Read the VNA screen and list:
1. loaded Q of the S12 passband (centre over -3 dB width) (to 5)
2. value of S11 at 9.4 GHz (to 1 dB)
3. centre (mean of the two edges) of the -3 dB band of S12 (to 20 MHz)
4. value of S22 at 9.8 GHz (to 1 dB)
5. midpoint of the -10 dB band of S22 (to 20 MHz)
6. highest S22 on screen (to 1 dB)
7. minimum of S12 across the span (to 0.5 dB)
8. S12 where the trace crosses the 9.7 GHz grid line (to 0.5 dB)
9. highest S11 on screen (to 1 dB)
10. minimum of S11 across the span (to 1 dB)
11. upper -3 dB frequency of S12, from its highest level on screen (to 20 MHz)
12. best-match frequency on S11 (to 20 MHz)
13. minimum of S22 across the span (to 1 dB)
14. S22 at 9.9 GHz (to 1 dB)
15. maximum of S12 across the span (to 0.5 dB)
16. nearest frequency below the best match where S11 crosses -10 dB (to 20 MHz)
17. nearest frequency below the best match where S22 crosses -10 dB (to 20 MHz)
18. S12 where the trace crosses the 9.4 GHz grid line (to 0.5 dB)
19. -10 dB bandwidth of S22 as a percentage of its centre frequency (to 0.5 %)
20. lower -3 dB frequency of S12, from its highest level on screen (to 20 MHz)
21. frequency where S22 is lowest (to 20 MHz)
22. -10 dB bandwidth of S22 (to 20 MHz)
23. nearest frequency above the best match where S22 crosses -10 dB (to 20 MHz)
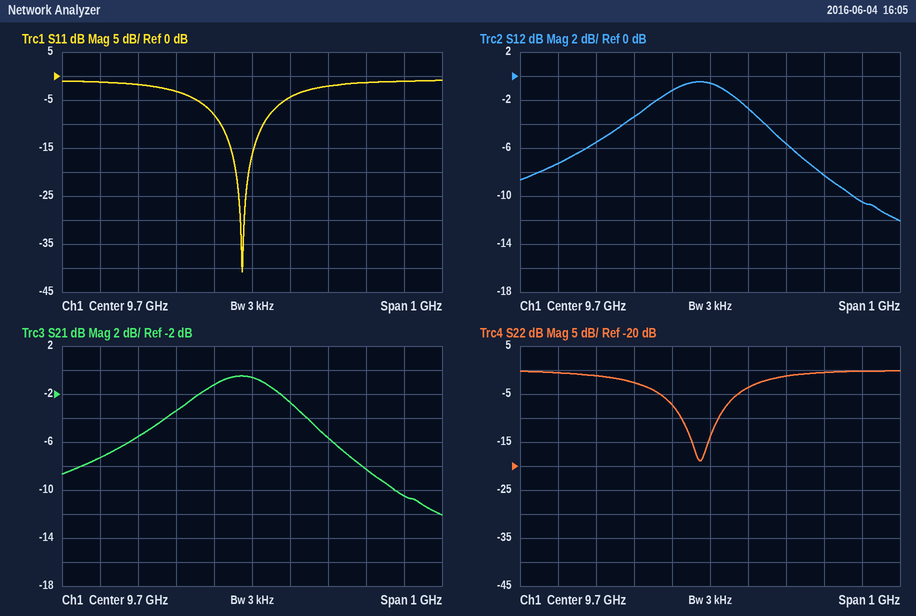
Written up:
30
-2 dB
9.66 GHz
-4 dB
9.68 GHz
0 dB
-12.0 dB
-0.5 dB
-1 dB
-41 dB
9.82 GHz
9.68 GHz
-19 dB
-1 dB
-0.5 dB
9.62 GHz
9.62 GHz
-5.5 dB
1.0 %
9.50 GHz
9.68 GHz
100 MHz
9.72 GHz
